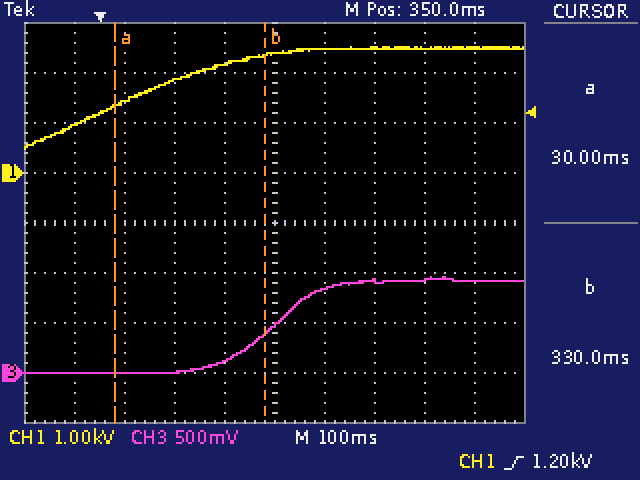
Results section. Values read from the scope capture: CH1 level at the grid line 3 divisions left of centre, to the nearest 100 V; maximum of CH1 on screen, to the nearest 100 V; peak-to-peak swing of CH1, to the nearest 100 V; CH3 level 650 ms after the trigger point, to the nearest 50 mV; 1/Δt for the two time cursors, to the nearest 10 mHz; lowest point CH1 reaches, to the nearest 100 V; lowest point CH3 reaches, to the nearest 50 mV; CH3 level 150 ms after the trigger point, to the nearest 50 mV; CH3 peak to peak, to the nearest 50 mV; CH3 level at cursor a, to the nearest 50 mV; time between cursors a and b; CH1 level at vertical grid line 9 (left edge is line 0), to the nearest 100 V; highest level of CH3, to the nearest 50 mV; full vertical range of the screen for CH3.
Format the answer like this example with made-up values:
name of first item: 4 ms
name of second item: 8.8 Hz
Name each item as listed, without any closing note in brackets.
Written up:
CH1 level at the grid line 3 divisions left of centre, to the nearest 100 V: 1.4 kV
maximum of CH1 on screen, to the nearest 100 V: 2.5 kV
peak-to-peak swing of CH1, to the nearest 100 V: 2.0 kV
CH3 level 650 ms after the trigger point, to the nearest 50 mV: 950 mV
1/Δt for the two time cursors, to the nearest 10 mHz: 3.33 Hz
lowest point CH1 reaches, to the nearest 100 V: 500 V
lowest point CH3 reaches, to the nearest 50 mV: 0 mV
CH3 level 150 ms after the trigger point, to the nearest 50 mV: 0 mV
CH3 peak to peak, to the nearest 50 mV: 950 mV
CH3 level at cursor a, to the nearest 50 mV: 0 mV
time between cursors a and b: 300 ms
CH1 level at vertical grid line 9 (left edge is line 0), to the nearest 100 V: 2.5 kV
highest level of CH3, to the nearest 50 mV: 950 mV
full vertical range of the screen for CH3: 4 V
